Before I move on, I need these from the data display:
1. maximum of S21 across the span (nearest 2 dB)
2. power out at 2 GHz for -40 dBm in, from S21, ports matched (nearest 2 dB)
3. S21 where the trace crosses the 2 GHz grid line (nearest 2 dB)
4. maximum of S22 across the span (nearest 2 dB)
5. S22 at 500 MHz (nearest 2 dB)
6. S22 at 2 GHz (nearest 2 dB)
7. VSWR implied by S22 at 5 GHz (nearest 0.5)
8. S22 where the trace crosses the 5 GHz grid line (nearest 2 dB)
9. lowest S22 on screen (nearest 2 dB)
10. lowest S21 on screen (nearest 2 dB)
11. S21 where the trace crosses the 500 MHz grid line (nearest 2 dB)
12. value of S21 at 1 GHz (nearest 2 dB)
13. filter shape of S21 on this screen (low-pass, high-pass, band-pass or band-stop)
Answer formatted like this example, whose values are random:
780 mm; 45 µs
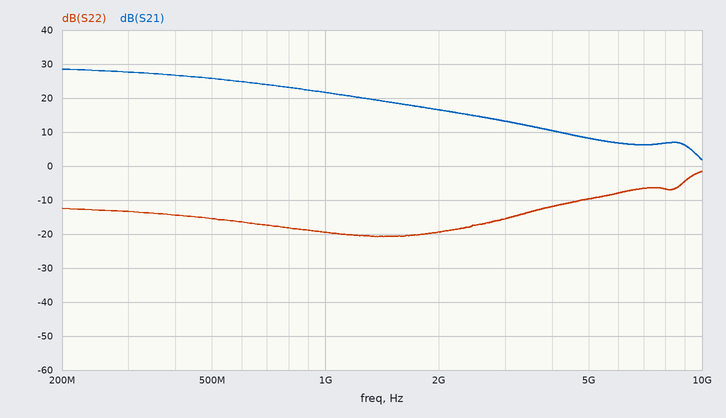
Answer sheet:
28 dB; -24 dBm; 16 dB; -2 dB; -16 dB; -20 dB; 2.0; -10 dB; -20 dB; 2 dB; 26 dB; 22 dB; low-pass
